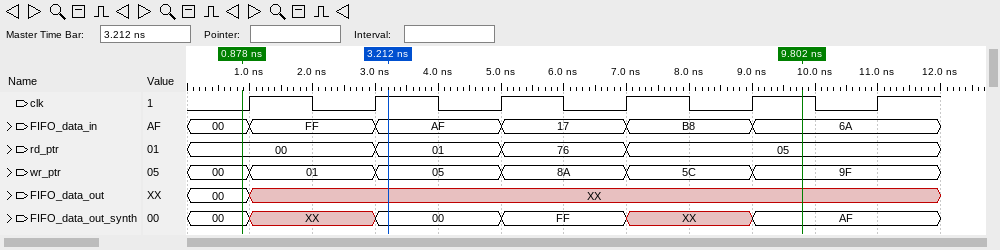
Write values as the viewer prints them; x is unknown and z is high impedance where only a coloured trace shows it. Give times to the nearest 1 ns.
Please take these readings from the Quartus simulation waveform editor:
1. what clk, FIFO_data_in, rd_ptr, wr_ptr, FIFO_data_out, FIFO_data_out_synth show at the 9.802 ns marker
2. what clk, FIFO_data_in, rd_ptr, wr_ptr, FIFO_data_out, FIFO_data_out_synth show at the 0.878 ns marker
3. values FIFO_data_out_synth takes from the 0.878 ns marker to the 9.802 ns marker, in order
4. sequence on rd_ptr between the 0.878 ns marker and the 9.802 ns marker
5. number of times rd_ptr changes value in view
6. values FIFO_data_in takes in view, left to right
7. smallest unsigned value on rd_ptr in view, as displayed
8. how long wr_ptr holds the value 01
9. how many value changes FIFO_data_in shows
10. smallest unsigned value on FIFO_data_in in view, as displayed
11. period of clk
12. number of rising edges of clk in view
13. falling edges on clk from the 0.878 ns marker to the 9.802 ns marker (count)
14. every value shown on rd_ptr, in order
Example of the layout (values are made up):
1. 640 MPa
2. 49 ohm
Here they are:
1. clk=1, FIFO_data_in=6A, rd_ptr=05, wr_ptr=9F, FIFO_data_out=XX, FIFO_data_out_synth=AF
2. clk=0, FIFO_data_in=00, rd_ptr=00, wr_ptr=00, FIFO_data_out=00, FIFO_data_out_synth=00
3. 00, XX, 00, FF, XX, AF
4. 00, 01, 76, 05
5. 3
6. 00, FF, AF, 17, B8, 6A
7. 00
8. 2 ns
9. 5
10. 00
11. 2 ns
12. 6
13. 4
14. 00, 01, 76, 05
